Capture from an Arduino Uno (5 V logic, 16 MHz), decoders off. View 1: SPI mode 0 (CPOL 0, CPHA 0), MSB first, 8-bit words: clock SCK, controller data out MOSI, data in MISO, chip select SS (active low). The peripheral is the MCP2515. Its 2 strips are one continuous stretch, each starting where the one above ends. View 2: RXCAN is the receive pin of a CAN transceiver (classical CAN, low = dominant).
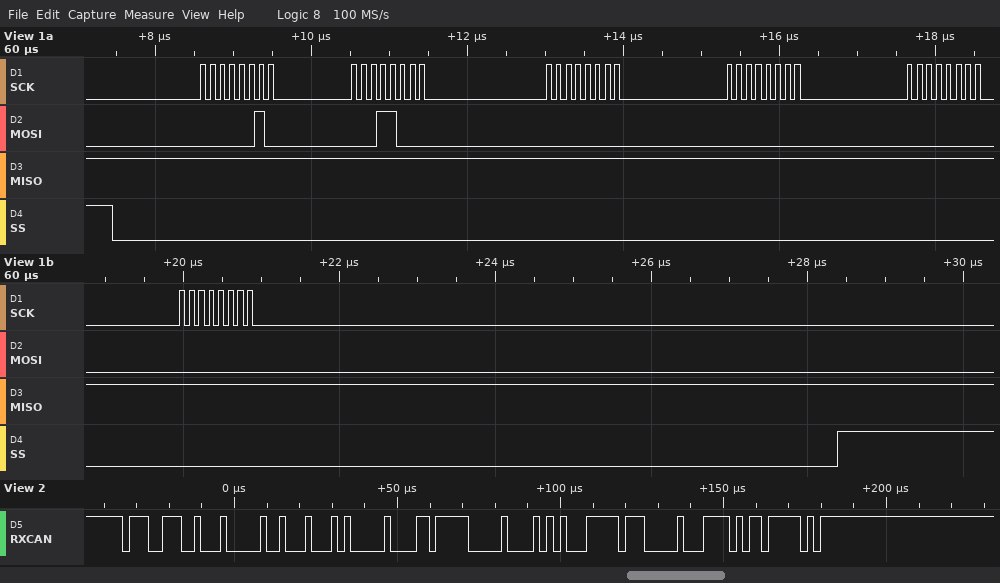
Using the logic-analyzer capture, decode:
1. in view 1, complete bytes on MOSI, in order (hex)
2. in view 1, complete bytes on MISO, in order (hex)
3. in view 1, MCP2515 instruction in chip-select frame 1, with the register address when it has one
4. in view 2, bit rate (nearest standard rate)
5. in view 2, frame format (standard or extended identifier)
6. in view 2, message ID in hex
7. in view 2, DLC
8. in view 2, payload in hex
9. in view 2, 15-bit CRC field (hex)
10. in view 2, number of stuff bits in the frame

02 18 00 00 00 00
FF FF FF FF FF FF
WRITE 0x18
500 kbit/s
standard
0x739
8
08 8A 00 DF 00 A8 FF 00
0x7ADF
7
